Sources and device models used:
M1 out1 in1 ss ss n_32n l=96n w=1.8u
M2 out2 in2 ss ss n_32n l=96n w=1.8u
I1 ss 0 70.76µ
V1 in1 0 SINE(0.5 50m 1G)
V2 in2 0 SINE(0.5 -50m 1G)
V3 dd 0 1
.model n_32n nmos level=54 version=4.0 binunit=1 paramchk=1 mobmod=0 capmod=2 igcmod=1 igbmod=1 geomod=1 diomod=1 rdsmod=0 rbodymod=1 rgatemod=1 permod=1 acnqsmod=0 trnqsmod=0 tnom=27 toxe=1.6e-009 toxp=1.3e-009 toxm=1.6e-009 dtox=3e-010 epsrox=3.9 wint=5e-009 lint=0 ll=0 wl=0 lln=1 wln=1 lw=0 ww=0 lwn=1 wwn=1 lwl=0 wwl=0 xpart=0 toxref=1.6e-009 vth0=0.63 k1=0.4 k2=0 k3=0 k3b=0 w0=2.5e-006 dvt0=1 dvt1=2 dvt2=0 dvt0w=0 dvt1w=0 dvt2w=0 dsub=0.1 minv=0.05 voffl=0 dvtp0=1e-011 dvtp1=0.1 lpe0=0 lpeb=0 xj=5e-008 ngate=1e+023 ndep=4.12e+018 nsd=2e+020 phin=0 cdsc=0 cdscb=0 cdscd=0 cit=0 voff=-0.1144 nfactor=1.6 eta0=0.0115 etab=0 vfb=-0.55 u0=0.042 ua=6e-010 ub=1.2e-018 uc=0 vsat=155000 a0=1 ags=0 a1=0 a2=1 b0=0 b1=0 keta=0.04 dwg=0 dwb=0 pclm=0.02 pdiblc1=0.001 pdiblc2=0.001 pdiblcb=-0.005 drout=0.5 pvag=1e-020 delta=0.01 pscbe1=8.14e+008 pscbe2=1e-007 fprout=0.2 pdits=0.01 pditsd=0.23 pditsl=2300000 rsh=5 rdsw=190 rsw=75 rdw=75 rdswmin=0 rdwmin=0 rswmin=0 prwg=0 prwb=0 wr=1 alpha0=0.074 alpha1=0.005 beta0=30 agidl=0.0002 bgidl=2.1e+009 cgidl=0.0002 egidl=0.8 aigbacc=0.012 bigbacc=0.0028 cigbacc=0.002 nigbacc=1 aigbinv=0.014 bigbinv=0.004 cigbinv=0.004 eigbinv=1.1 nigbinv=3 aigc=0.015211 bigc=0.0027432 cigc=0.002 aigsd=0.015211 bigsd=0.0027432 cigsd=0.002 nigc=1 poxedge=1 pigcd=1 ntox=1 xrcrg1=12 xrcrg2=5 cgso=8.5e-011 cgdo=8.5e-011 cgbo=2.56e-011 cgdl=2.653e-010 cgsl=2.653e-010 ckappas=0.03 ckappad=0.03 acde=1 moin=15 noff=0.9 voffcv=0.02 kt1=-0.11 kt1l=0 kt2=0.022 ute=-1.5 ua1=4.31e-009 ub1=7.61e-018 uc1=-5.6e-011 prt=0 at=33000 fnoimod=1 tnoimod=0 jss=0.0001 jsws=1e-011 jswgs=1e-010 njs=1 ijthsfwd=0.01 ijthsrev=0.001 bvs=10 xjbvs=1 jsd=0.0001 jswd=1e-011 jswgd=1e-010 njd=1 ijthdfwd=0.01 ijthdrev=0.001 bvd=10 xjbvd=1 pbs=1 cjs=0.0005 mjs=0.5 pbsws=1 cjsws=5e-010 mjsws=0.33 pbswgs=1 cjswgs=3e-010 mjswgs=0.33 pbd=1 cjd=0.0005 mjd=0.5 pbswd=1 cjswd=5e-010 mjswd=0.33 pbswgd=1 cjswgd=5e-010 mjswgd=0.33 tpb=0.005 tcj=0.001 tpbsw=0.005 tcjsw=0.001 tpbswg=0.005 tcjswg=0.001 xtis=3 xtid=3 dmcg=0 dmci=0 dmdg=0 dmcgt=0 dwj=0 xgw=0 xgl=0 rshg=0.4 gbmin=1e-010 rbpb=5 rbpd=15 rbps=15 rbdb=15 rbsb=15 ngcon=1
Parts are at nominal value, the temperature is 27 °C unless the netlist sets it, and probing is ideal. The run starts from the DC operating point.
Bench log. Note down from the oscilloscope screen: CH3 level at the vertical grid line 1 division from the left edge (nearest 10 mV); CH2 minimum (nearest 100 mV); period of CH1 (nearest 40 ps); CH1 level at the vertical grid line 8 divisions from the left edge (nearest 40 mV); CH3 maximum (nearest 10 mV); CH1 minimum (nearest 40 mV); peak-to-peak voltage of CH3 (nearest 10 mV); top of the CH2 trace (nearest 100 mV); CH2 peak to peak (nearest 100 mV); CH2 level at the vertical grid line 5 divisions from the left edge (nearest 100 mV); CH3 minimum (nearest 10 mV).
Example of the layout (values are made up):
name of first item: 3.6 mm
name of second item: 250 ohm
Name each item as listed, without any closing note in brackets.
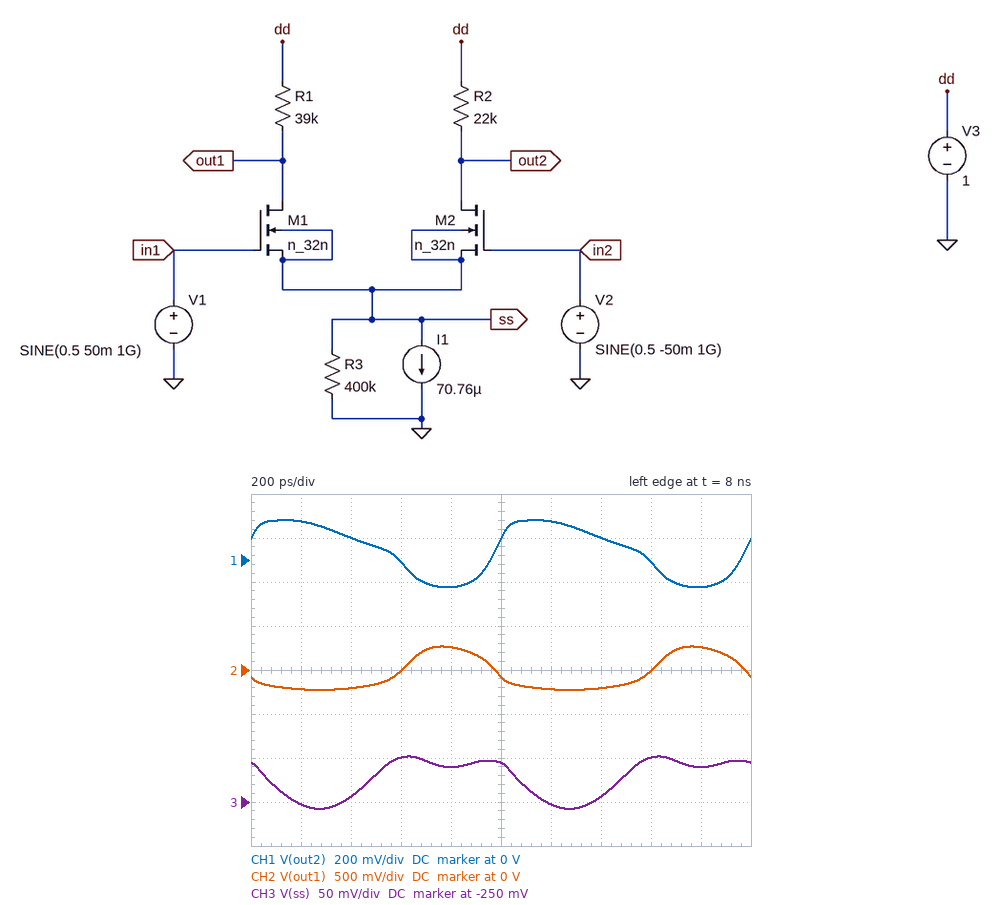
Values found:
CH3 level at the vertical grid line 1 division from the left edge: -250 mV
CH2 minimum: -200 mV
period of CH1: 1.00 ns
CH1 level at the vertical grid line 8 divisions from the left edge: 0 V
CH3 maximum: -200 mV
CH1 minimum: -120 mV
peak-to-peak voltage of CH3: 60 mV
top of the CH2 trace: 300 mV
CH2 peak to peak: 500 mV
CH2 level at the vertical grid line 5 divisions from the left edge: -100 mV
CH3 minimum: -260 mV
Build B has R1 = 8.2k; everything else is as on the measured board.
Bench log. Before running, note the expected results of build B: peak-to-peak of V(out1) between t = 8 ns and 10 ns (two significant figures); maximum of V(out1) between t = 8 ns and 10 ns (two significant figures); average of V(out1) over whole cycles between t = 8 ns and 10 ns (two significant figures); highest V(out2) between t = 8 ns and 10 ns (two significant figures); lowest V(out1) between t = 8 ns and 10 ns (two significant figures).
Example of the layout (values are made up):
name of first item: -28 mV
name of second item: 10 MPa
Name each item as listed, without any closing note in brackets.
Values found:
peak-to-peak of V(out1) between t = 8 ns and 10 ns: 310 mV
maximum of V(out1) between t = 8 ns and 10 ns: 840 mV
average of V(out1) over whole cycles between t = 8 ns and 10 ns: 700 mV
highest V(out2) between t = 8 ns and 10 ns: 710 mV
lowest V(out1) between t = 8 ns and 10 ns: 530 mV
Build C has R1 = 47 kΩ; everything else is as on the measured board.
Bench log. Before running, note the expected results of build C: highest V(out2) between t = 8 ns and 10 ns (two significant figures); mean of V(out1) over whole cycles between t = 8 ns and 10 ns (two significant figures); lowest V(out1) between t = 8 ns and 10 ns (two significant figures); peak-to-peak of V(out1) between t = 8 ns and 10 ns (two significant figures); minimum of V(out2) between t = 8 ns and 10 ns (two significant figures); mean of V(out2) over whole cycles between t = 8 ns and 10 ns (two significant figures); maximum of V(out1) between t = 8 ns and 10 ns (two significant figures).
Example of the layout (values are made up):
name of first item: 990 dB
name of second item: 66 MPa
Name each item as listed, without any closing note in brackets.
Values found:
highest V(out2) between t = 8 ns and 10 ns: 77 mV
mean of V(out1) over whole cycles between t = 8 ns and 10 ns: -120 mV
lowest V(out1) between t = 8 ns and 10 ns: -240 mV
peak-to-peak of V(out1) between t = 8 ns and 10 ns: 360 mV
minimum of V(out2) between t = 8 ns and 10 ns: -130 mV
mean of V(out2) over whole cycles between t = 8 ns and 10 ns: -22 mV
maximum of V(out1) between t = 8 ns and 10 ns: 120 mV
